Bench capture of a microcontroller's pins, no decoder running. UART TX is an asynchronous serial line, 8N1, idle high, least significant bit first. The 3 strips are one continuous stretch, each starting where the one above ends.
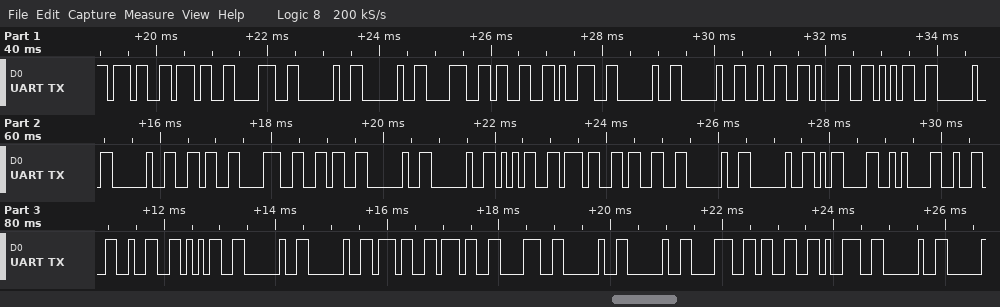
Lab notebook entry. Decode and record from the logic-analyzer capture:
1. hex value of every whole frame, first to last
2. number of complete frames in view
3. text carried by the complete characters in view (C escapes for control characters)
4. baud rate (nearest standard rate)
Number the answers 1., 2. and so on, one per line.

1. 37 37 38 20 20 38 33 39 20 20 32 31 35 20 20 36 38 36 20 20 35 37 33 20 20 0D 0A 32 32 35 20 20 37 37 38 20 20 38 33 39 20
2. 41
3. "778  839  215  686  573  \r\n225  778  839 "
4. 9600 baud
